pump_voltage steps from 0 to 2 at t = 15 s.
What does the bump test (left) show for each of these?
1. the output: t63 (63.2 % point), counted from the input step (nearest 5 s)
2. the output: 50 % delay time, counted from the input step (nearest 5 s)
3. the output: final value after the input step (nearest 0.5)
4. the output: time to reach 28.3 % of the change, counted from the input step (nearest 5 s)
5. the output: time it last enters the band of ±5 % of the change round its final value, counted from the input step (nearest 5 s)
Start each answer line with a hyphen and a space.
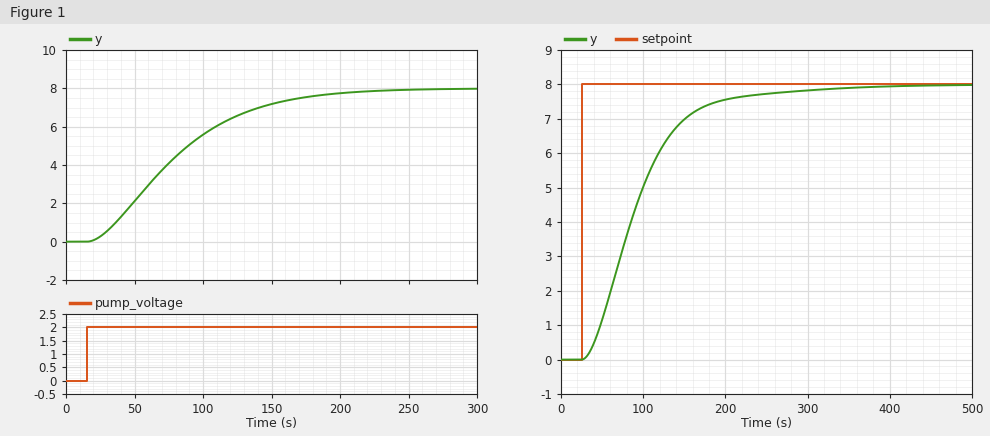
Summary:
- 75 s
- 60 s
- 8.0
- 35 s
- 165 s
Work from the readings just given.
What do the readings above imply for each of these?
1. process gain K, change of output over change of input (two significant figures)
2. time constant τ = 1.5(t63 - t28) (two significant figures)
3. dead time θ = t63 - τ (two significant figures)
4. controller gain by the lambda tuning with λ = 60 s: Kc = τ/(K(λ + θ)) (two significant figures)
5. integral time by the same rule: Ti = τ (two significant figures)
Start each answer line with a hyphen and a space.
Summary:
- 4.0
- 60 s
- 15 s
- 0.20
- 60 s
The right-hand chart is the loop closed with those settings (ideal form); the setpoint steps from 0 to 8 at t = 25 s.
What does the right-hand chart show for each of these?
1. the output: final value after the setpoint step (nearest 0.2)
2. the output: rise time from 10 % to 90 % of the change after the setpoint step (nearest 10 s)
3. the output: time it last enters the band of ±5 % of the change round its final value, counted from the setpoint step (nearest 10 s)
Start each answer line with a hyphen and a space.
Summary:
- 8.0
- 120 s
- 180 s
